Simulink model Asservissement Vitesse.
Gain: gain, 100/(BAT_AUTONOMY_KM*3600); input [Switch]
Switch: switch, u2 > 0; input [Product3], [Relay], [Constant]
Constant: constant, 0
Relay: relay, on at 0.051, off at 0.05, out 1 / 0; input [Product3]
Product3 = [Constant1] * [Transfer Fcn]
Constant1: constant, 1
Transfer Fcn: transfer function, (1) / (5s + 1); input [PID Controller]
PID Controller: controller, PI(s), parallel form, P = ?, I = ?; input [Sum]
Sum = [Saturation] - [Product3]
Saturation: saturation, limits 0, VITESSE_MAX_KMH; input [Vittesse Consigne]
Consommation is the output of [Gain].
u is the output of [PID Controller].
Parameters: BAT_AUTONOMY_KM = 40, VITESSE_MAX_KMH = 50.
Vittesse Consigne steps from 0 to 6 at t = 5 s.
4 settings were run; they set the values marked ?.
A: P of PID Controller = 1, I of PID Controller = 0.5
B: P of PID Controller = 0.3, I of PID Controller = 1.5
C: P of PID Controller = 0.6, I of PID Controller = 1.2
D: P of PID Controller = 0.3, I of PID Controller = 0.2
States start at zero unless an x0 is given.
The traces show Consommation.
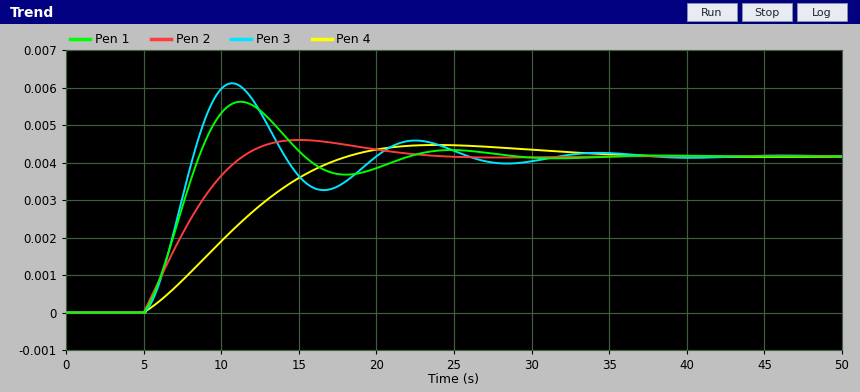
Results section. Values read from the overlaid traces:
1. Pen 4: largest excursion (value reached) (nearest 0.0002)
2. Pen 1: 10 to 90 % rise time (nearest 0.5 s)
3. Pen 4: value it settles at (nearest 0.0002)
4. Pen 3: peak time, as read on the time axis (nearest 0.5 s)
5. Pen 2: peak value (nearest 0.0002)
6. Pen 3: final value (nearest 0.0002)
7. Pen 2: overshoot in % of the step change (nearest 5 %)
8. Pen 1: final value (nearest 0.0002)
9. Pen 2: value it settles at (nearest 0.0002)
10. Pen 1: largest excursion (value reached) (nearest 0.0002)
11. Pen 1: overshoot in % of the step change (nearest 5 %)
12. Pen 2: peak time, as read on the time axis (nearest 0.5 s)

0.0044
2.5 s
0.0042
10.5 s
0.0046
0.0042
10 %
0.0042
0.0042
0.0056
35 %
15.0 s
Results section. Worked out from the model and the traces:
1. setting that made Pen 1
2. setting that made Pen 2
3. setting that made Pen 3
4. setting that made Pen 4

C
A
B
D
